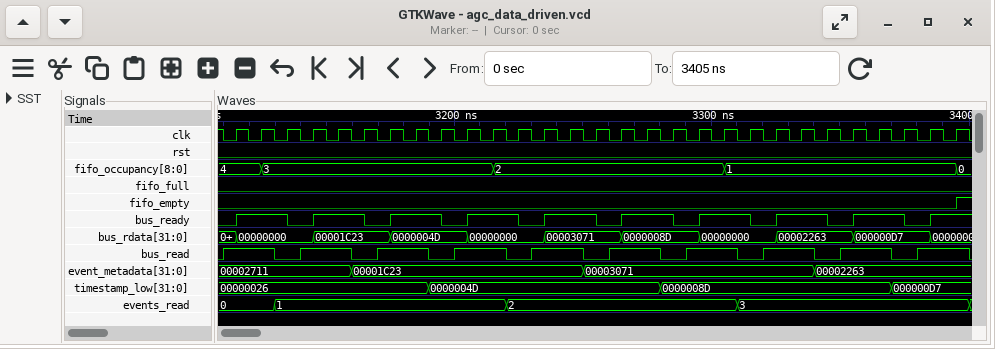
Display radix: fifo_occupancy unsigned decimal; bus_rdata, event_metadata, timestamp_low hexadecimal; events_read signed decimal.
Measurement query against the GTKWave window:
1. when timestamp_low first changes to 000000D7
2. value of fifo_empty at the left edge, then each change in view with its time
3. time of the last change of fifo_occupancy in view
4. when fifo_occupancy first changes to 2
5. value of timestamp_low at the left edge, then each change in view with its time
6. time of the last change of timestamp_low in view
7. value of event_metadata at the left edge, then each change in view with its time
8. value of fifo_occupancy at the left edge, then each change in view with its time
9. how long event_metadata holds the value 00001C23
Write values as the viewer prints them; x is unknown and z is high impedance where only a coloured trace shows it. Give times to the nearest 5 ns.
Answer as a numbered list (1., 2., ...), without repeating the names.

1. 3370 ns
2. 0, 1 at 3395 ns
3. 3395 ns
4. 3215 ns
5. 00000026, 0000004D at 3190 ns, 0000008D at 3280 ns, 000000D7 at 3370 ns
6. 3370 ns
7. 00002711, 00001C23 at 3160 ns, 00003071 at 3250 ns, 00002263 at 3340 ns
8. 4, 3 at 3125 ns, 2 at 3215 ns, 1 at 3305 ns, 0 at 3395 ns
9. 90 ns
